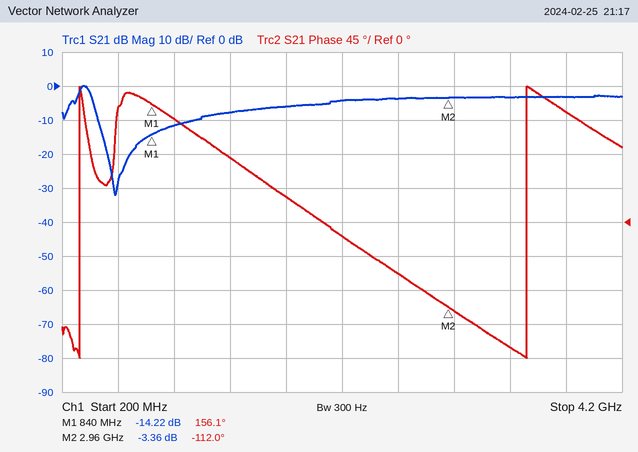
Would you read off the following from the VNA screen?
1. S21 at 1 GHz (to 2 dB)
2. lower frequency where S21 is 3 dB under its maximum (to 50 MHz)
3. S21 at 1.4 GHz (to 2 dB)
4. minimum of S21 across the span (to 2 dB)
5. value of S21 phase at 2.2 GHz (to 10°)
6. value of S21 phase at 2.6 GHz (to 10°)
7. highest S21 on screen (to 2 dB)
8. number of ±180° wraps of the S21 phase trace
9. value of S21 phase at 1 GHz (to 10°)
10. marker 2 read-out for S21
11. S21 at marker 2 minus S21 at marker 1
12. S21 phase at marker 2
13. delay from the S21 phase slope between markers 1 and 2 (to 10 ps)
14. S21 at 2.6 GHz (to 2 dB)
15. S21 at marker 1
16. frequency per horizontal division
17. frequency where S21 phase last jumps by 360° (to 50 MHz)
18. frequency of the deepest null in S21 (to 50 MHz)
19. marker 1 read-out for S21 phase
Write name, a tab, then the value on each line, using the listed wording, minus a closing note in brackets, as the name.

S21 at 1 GHz	-12 dB
lower frequency where S21 is 3 dB under its maximum	300 MHz
S21 at 1.4 GHz	-8 dB
minimum of S21 across the span	-32 dB
value of S21 phase at 2.2 GHz	-20°
value of S21 phase at 2.6 GHz	-70°
highest S21 on screen	0 dB
number of ±180° wraps of the S21 phase trace	2
value of S21 phase at 1 GHz	140°
marker 2 read-out for S21	-3.36 dB
S21 at marker 2 minus S21 at marker 1	10.86 dB
S21 phase at marker 2	-112.0°
delay from the S21 phase slope between markers 1 and 2	350 ps
S21 at 2.6 GHz	-4 dB
S21 at marker 1	-14.22 dB
frequency per horizontal division	400 MHz
frequency where S21 phase last jumps by 360°	3.50 GHz
frequency of the deepest null in S21	600 MHz
marker 1 read-out for S21 phase	156.1°
